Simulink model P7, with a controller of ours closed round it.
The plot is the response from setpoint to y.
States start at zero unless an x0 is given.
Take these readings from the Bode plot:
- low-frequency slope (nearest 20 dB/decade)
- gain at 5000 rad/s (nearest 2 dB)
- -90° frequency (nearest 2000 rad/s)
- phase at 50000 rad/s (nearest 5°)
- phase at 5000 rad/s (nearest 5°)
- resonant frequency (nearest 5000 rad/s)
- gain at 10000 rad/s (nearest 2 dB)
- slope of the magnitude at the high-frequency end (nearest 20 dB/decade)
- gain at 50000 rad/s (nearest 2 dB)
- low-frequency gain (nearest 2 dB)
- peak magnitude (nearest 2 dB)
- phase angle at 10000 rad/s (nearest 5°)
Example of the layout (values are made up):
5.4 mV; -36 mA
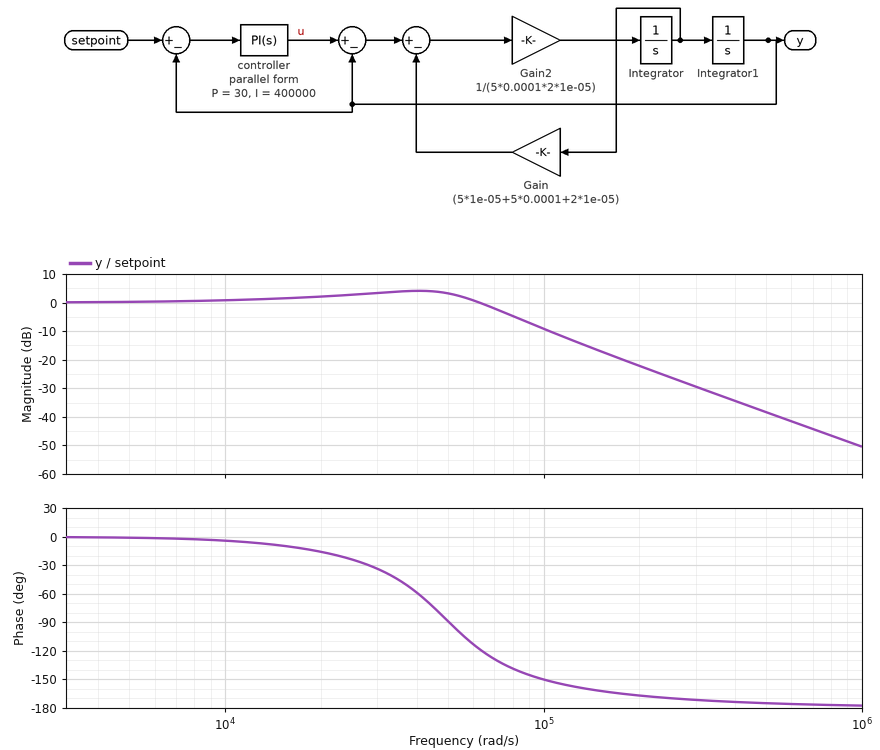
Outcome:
0 dB/decade; 0 dB; 50000 rad/s; -90°; 0°; 40000 rad/s; 0 dB; -40 dB/decade; 4 dB; 0 dB; 4 dB; -5°
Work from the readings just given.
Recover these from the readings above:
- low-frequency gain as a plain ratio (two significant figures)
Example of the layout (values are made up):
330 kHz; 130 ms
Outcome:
1.0
